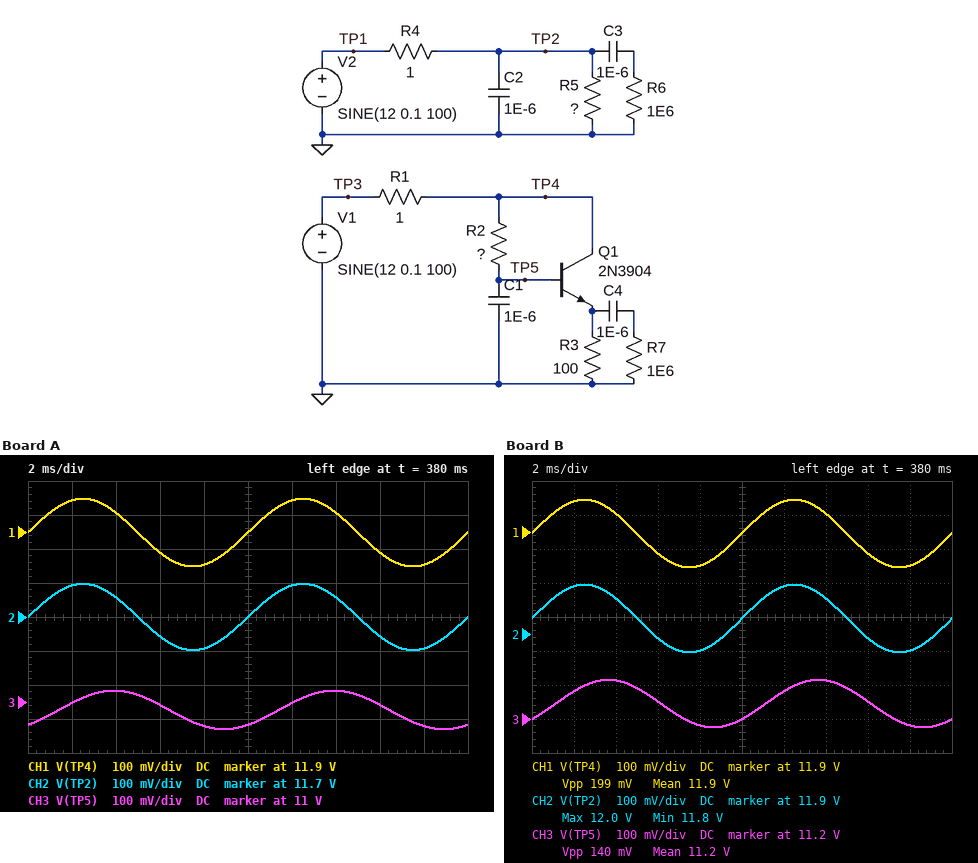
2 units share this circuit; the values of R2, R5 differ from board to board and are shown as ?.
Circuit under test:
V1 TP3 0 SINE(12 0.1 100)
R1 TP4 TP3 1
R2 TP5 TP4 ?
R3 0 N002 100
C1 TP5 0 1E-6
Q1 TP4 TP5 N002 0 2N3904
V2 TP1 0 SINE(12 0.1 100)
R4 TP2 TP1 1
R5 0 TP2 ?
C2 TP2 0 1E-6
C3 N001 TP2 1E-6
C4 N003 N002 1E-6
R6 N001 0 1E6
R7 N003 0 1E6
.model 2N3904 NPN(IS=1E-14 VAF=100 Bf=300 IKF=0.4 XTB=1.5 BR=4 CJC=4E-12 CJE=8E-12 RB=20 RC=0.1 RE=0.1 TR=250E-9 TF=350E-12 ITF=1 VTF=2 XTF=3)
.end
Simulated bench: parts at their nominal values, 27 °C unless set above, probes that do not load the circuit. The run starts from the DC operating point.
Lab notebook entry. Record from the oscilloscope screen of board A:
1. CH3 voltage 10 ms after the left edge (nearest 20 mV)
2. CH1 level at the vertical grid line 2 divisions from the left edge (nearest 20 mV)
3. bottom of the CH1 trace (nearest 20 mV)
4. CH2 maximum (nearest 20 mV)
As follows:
10.94 V
11.96 V
11.80 V
11.80 V
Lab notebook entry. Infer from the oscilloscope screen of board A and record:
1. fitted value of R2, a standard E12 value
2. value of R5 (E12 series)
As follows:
2.2 kΩ
39 Ω
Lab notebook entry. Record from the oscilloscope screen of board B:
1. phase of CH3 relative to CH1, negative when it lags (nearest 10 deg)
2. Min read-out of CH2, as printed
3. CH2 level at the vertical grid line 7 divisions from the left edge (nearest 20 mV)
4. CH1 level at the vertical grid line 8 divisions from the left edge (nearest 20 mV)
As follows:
-40 deg
11.8 V
12.00 V
11.84 V
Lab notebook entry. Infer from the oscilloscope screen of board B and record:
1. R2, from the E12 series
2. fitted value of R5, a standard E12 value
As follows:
1.5 kΩ
220 Ω
